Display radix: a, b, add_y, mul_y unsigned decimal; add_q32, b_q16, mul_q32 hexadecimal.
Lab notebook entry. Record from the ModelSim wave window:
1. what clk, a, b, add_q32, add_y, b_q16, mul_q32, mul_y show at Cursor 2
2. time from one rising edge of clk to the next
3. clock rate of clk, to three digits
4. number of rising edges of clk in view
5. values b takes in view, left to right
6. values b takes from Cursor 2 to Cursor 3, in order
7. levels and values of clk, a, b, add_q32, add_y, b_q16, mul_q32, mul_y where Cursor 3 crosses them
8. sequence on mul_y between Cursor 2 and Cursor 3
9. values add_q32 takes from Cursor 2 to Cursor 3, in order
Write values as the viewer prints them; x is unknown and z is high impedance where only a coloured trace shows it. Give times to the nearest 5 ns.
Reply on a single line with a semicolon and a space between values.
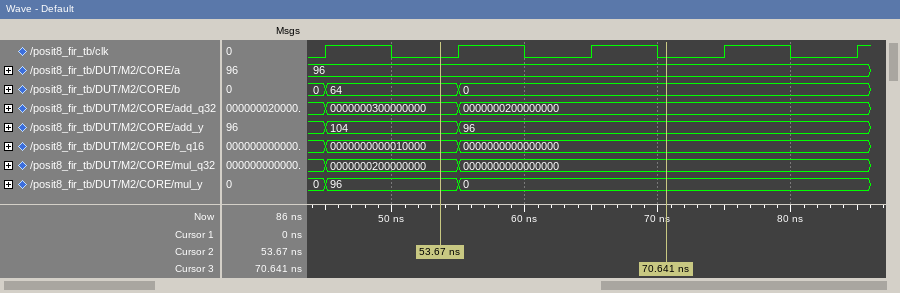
clk=0, a=96, b=64, add_q32=0000000300000000, add_y=104, b_q16=0000000000010000, mul_q32=0000000200000000, mul_y=96; 10 ns; 100 MHz; 5; 0, 64, 0; 64, 0; clk=0, a=96, b=0, add_q32=0000000200000000, add_y=96, b_q16=0000000000000000, mul_q32=0000000000000000, mul_y=0; 96, 0; 0000000300000000, 0000000200000000
